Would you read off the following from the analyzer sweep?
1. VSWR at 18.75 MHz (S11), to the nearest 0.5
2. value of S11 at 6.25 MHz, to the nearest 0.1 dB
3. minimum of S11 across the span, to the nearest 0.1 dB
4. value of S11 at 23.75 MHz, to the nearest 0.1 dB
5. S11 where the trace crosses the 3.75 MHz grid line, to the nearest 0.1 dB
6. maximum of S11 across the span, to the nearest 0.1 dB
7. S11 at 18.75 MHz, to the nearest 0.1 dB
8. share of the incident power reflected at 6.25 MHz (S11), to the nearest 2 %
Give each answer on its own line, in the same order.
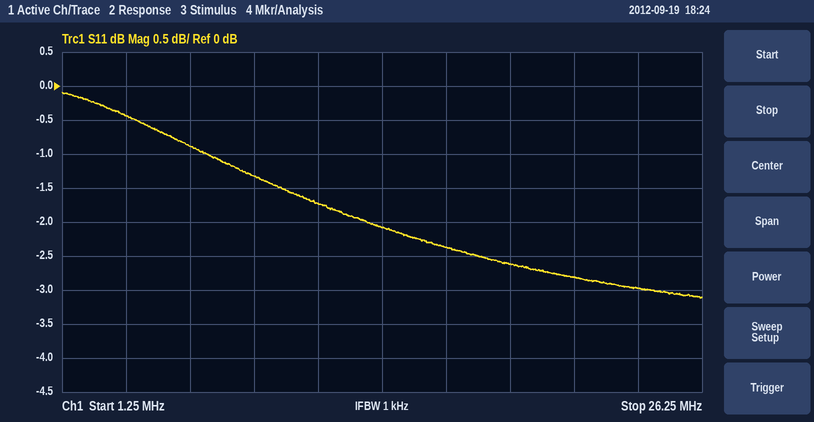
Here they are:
6.5
-0.9 dB
-3.1 dB
-3.0 dB
-0.4 dB
-0.1 dB
-2.6 dB
82 %
